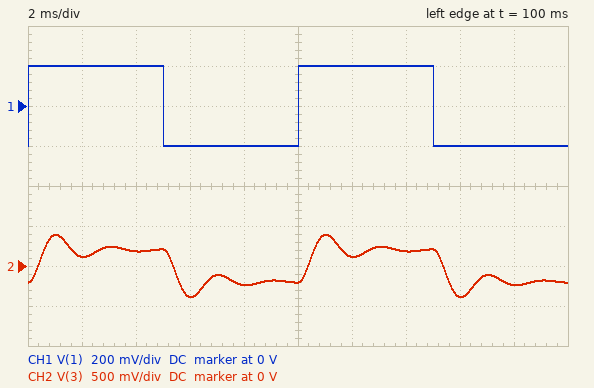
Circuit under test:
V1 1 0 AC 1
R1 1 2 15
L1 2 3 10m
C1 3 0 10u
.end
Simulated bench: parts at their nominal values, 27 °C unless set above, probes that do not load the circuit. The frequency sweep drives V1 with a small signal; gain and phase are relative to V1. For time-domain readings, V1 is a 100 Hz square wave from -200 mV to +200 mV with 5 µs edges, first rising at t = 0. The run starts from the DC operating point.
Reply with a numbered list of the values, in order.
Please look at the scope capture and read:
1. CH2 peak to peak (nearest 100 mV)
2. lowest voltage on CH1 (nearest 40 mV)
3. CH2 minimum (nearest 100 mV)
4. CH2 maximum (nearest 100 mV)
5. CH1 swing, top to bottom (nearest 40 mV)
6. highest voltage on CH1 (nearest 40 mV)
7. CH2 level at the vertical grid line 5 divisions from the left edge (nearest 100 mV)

1. 800 mV
2. -200 mV
3. -400 mV
4. 400 mV
5. 400 mV
6. 200 mV
7. -200 mV
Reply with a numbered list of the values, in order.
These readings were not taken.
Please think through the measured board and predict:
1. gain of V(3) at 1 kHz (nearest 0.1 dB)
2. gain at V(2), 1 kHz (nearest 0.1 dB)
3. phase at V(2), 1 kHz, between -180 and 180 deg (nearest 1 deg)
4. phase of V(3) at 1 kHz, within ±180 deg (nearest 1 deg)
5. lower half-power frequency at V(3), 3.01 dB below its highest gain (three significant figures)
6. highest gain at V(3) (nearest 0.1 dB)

1. -9.8 dB
2. -0.4 dB
3. 18 deg
4. -162 deg
5. 329 Hz
6. 6.7 dB
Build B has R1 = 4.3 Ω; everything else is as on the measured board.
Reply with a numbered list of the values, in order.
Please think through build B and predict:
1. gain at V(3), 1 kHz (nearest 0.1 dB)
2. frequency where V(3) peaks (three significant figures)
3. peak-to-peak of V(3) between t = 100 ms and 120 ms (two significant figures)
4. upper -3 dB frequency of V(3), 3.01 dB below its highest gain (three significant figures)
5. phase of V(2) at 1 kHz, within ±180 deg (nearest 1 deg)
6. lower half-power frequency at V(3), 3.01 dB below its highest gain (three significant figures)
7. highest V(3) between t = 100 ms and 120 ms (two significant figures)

1. -9.4 dB
2. 501 Hz
3. 1.4 V
4. 534 Hz
5. 5 deg
6. 465 Hz
7. 690 mV
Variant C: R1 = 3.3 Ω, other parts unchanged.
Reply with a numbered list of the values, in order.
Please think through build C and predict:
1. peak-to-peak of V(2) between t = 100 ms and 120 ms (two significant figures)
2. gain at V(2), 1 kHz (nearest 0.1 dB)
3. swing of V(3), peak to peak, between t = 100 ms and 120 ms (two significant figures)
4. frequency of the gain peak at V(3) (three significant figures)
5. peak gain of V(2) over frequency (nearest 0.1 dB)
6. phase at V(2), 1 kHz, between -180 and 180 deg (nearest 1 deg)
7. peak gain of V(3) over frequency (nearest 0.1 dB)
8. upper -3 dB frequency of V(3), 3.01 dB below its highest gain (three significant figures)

1. 520 mV
2. 0 dB
3. 1.6 V
4. 502 Hz
5. 0 dB
6. 4 deg
7. 19.6 dB
8. 528 Hz
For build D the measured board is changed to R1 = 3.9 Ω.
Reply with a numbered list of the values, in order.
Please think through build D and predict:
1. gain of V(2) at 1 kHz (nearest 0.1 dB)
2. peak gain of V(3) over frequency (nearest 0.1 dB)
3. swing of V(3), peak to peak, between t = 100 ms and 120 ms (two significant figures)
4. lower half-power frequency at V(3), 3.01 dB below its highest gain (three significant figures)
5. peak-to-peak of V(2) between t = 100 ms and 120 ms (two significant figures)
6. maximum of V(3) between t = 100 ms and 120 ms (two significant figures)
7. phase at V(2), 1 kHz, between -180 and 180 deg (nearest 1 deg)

1. 0 dB
2. 18.2 dB
3. 1.5 V
4. 469 Hz
5. 520 mV
6. 730 mV
7. 5 deg
